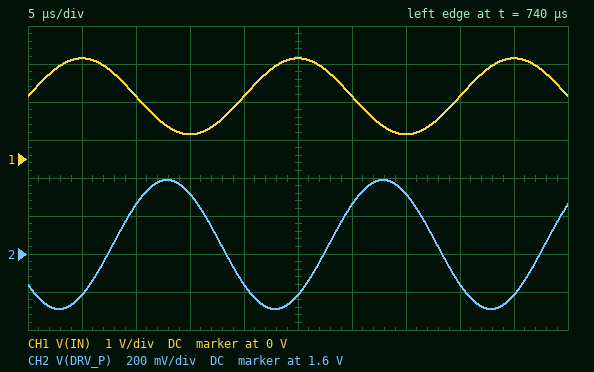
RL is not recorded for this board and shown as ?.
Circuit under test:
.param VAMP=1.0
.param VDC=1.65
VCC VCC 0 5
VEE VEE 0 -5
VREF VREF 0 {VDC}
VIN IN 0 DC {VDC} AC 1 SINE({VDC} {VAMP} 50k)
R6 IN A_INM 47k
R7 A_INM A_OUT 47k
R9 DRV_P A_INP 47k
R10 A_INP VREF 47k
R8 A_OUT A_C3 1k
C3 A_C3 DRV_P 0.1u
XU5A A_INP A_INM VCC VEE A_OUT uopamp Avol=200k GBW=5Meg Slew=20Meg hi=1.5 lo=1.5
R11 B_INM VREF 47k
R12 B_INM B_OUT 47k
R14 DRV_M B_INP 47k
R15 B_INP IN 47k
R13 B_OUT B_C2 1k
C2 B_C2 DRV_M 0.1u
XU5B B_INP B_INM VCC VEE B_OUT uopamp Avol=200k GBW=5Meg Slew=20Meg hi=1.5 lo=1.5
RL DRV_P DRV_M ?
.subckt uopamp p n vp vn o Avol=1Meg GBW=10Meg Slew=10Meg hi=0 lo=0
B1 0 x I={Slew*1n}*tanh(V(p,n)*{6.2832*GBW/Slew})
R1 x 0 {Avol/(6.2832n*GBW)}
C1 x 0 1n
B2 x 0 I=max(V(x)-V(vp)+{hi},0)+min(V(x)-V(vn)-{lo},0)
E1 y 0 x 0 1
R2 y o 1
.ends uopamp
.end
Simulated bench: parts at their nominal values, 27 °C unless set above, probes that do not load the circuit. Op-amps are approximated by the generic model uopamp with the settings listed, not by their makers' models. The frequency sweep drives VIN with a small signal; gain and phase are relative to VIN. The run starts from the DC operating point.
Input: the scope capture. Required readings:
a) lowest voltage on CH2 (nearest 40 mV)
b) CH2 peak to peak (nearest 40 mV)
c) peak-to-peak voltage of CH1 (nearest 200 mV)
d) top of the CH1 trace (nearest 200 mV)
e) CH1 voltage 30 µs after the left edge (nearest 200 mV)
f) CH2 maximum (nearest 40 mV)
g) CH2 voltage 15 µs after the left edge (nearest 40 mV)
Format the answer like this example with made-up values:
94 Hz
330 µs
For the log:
1.32 V
680 mV
2.0 V
2.6 V
1.6 V
2.00 V
1.92 V
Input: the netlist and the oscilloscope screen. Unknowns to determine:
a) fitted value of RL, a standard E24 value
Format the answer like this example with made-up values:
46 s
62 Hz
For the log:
750 Ω
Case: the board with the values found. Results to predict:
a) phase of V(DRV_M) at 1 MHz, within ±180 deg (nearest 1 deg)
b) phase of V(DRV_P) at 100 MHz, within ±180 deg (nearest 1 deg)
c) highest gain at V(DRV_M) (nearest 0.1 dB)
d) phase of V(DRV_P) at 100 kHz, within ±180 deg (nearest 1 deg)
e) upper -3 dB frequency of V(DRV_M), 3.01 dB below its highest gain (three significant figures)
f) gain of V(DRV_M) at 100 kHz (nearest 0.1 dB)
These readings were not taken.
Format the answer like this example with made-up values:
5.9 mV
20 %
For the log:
-30 deg
61 deg
-1.4 dB
-162 deg
35.1 kHz
-7.3 dB
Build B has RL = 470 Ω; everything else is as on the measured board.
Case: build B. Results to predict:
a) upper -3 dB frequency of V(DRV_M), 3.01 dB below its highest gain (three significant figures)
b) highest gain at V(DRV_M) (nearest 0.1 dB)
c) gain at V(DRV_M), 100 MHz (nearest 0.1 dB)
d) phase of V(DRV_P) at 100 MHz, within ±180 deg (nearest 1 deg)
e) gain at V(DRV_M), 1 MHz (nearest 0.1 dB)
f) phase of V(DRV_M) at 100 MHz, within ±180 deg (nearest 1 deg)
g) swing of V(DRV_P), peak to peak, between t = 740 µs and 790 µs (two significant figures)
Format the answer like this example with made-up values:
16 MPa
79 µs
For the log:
30.6 kHz
-2.8 dB
-41.9 dB
48 deg
-13.1 dB
-37 deg
490 mV
